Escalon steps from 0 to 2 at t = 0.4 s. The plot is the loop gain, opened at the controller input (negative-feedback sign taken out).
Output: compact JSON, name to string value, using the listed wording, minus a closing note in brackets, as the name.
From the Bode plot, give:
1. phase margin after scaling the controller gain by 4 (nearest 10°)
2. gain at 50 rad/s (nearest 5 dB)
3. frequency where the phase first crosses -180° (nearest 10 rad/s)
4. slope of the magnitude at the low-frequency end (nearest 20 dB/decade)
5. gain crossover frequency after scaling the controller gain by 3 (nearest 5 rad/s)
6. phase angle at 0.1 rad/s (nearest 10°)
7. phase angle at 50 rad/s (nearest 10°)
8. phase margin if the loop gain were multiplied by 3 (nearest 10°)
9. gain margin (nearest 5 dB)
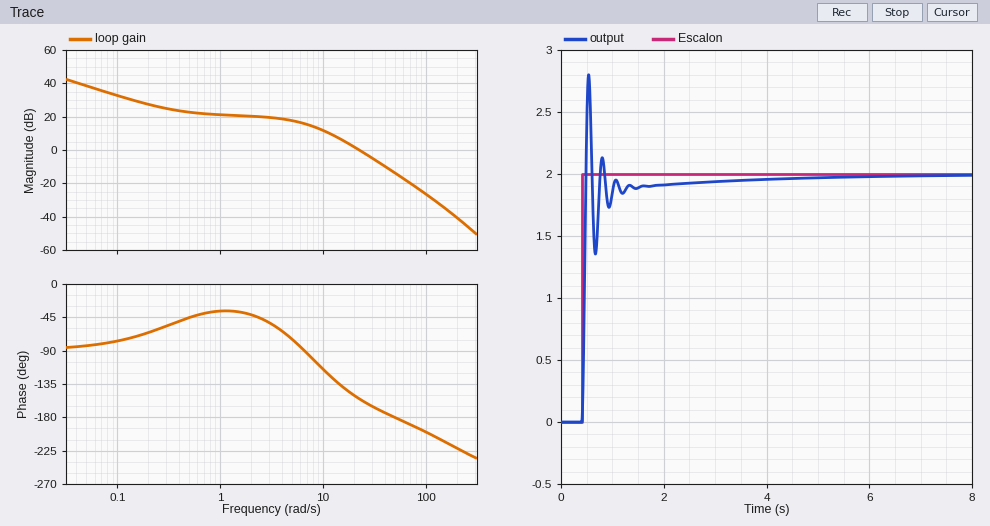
{"phase margin after scaling the controller gain by 4": "0°", "gain at 50 rad/s": "-15 dB", "frequency where the phase first crosses -180°": "50 rad/s", "slope of the magnitude at the low-frequency end": "-20 dB/decade", "gain crossover frequency after scaling the controller gain by 3": "40 rad/s", "phase angle at 0.1 rad/s": "-80°", "phase angle at 50 rad/s": "-180°", "phase margin if the loop gain were multiplied by 3": "10°", "gain margin": "15 dB"}
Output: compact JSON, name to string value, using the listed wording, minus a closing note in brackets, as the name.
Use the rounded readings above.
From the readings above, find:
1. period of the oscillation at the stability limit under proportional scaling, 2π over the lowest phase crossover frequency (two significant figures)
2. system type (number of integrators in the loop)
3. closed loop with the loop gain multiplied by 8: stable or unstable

{"period of the oscillation at the stability limit under proportional scaling, 2π over the lowest phase crossover frequency": "0.13 s", "system type": "1", "closed loop with the loop gain multiplied by 8: stable or unstable": "unstable"}
